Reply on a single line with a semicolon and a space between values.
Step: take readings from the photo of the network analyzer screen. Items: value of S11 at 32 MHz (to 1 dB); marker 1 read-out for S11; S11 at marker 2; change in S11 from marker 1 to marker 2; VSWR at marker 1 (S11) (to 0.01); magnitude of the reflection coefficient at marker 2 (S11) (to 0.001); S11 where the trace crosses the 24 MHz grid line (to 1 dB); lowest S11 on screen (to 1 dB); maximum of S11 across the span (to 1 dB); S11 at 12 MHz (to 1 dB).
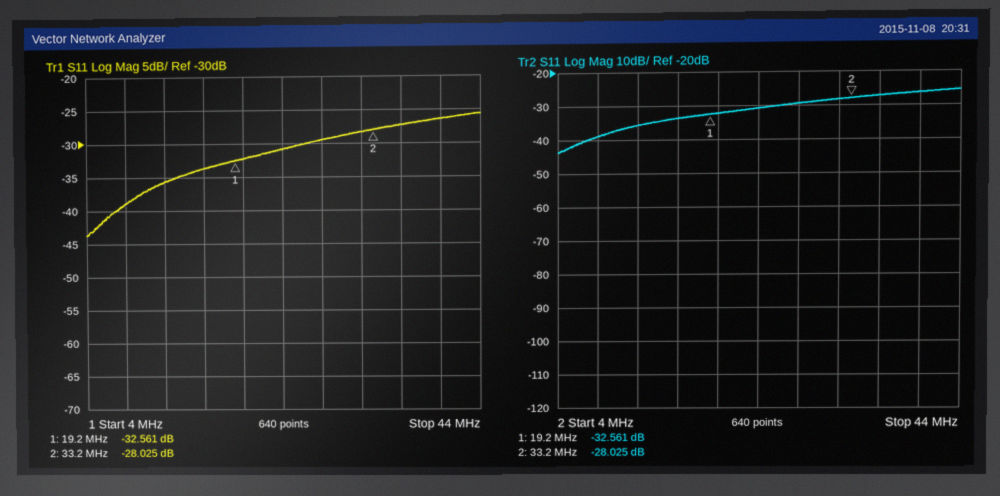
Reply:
-28 dB; -32.561 dB; -28.025 dB; 4.536 dB; 1.05; 0.040; -31 dB; -44 dB; -26 dB; -36 dB
